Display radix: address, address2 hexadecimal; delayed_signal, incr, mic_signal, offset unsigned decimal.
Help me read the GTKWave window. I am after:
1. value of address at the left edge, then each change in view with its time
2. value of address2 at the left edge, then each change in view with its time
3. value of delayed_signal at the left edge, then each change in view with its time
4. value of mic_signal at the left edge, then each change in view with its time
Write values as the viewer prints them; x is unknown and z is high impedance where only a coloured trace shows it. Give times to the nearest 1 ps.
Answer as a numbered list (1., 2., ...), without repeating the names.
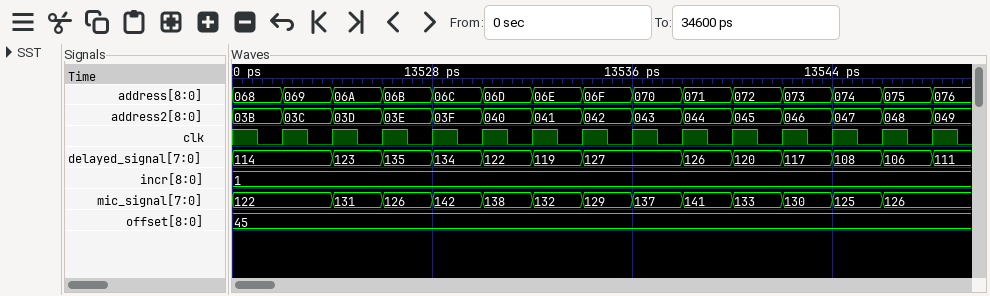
1. 068, 069 at 13522 ps, 06A at 13524 ps, 06B at 13526 ps, 06C at 13528 ps, 06D at 13530 ps, 06E at 13532 ps, 06F at 13534 ps, 070 at 13536 ps, 071 at 13538 ps, 072 at 13540 ps, 073 at 13542 ps, 074 at 13544 ps, 075 at 13546 ps, 076 at 13548 ps
2. 03B, 03C at 13522 ps, 03D at 13524 ps, 03E at 13526 ps, 03F at 13528 ps, 040 at 13530 ps, 041 at 13532 ps, 042 at 13534 ps, 043 at 13536 ps, 044 at 13538 ps, 045 at 13540 ps, 046 at 13542 ps, 047 at 13544 ps, 048 at 13546 ps, 049 at 13548 ps
3. 114, 123 at 13524 ps, 135 at 13526 ps, 134 at 13528 ps, 122 at 13530 ps, 119 at 13532 ps, 127 at 13534 ps, 126 at 13538 ps, 120 at 13540 ps, 117 at 13542 ps, 108 at 13544 ps, 106 at 13546 ps, 111 at 13548 ps
4. 122, 131 at 13524 ps, 126 at 13526 ps, 142 at 13528 ps, 138 at 13530 ps, 132 at 13532 ps, 129 at 13534 ps, 137 at 13536 ps, 141 at 13538 ps, 133 at 13540 ps, 130 at 13542 ps, 125 at 13544 ps, 126 at 13546 ps
